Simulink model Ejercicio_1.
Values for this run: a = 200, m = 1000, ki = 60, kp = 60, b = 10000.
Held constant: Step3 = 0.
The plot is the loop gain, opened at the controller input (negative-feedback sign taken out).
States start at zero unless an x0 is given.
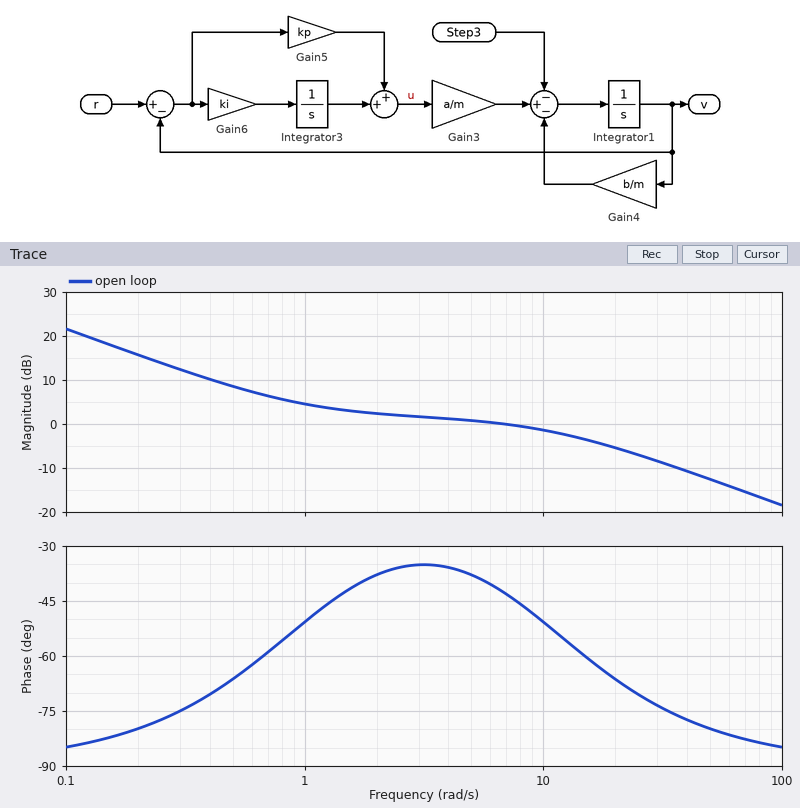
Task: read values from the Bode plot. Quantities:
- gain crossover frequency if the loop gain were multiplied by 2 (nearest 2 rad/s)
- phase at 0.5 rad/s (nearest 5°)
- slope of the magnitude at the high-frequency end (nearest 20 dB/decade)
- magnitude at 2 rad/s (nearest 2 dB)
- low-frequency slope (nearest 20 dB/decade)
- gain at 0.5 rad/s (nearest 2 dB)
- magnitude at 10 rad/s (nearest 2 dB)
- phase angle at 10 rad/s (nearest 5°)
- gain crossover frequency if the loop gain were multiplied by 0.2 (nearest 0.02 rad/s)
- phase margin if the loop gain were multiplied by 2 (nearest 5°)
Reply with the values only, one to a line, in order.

22 rad/s
-65°
-20 dB/decade
2 dB
-20 dB/decade
8 dB
-2 dB
-50°
0.24 rad/s
110°
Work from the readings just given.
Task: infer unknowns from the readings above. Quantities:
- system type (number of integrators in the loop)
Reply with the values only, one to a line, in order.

1
